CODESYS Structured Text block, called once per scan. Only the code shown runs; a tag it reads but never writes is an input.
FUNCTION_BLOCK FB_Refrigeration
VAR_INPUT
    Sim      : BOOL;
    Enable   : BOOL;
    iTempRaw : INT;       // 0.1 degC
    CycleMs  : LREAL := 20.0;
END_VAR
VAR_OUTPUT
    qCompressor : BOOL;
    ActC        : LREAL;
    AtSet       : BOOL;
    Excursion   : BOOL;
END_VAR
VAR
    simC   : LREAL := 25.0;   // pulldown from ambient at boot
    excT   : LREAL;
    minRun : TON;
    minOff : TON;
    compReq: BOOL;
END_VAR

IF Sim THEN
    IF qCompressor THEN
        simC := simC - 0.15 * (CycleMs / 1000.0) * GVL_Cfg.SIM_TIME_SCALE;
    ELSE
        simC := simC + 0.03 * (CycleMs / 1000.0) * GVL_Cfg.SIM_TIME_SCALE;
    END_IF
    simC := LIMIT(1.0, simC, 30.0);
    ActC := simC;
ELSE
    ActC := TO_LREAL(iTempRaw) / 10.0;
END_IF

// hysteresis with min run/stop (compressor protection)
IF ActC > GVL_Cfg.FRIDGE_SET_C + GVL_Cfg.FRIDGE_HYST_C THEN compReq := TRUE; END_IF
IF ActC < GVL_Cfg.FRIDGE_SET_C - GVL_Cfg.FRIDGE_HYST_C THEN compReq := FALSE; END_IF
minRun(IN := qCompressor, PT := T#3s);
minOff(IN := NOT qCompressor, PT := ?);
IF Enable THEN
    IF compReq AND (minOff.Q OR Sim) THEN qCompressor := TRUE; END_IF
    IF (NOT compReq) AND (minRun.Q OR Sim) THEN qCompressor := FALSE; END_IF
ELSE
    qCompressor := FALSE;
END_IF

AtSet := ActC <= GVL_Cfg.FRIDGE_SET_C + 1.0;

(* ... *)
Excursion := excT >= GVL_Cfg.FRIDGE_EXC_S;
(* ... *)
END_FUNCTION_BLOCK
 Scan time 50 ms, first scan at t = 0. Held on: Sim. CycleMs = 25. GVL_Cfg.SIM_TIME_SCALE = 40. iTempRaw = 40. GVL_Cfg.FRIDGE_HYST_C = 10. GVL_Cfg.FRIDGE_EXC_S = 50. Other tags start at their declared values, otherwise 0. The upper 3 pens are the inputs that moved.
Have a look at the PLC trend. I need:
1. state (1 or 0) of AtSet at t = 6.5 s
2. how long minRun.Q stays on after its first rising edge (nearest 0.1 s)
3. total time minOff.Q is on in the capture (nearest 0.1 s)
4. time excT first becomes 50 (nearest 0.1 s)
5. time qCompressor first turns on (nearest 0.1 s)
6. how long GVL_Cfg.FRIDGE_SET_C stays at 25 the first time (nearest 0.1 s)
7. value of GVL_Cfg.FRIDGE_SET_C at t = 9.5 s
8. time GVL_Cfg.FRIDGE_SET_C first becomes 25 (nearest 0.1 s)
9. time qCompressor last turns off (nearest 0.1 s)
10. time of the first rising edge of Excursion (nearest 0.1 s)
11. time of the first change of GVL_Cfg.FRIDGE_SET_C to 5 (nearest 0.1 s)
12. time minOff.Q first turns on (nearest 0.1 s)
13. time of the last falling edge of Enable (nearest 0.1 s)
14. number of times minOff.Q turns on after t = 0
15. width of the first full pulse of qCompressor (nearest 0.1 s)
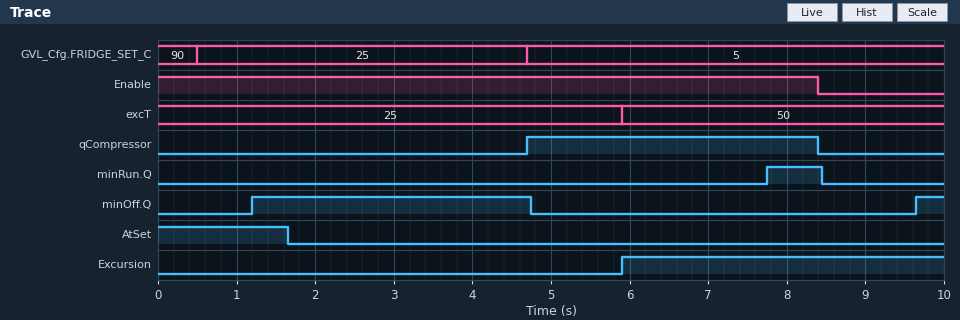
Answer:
0
0.7 s
3.9 s
5.9 s
4.7 s
4.2 s
5
0.5 s
8.4 s
5.9 s
4.7 s
1.2 s
8.4 s
2
3.7 s
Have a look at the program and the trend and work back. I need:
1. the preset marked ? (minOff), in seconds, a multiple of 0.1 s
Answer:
1.2 s
